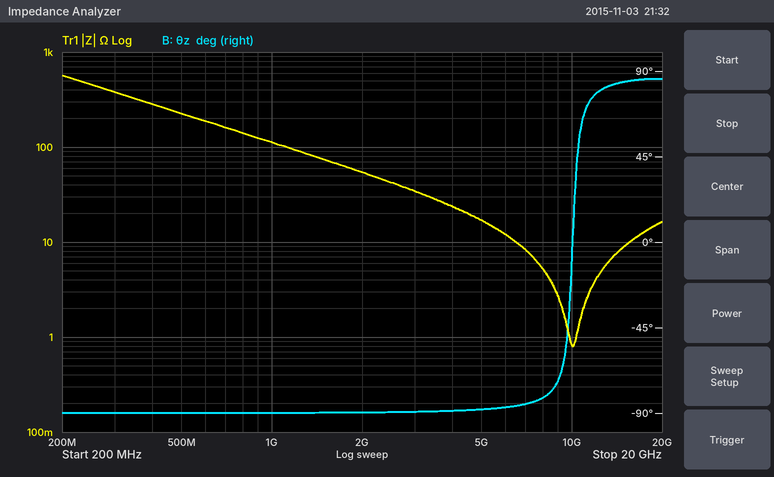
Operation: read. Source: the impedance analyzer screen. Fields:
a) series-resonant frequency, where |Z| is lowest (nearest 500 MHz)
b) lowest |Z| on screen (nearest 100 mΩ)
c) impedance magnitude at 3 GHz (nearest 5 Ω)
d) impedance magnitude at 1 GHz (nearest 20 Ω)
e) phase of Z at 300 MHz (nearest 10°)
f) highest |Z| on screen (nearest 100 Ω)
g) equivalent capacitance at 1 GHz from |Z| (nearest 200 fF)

10.0 GHz
800 mΩ
35 Ω
120 Ω
-90°
600 Ω
1.4 pF
